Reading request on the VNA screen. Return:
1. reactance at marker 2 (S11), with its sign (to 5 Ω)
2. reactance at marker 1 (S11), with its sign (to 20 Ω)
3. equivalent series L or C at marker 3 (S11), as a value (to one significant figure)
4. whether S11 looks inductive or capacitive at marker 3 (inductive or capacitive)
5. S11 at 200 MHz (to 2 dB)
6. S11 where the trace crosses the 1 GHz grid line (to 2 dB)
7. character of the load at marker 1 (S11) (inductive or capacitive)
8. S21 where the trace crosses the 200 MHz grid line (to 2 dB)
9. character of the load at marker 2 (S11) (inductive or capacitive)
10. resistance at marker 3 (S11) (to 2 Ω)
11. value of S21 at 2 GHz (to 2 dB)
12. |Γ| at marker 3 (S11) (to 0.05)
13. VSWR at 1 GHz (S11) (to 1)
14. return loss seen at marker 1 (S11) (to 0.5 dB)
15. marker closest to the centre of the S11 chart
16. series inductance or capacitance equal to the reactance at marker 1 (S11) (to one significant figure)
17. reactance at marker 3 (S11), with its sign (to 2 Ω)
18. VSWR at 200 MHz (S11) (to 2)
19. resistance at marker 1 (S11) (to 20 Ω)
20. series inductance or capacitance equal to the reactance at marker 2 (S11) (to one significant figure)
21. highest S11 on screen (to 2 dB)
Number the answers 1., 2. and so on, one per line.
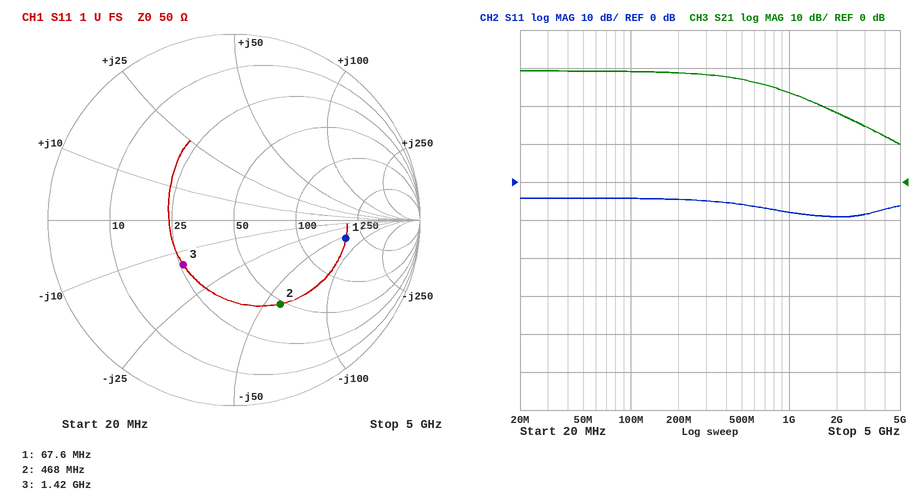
1. -60 Ω
2. -60 Ω
3. 8 pF
4. capacitive
5. -4 dB
6. -8 dB
7. capacitive
8. 28 dB
9. capacitive
10. 26 Ω
11. 18 dB
12. 0.35
13. 2
14. 4.5 dB
15. marker 3
16. 40 pF
17. -14 Ω
18. 4
19. 180 Ω
20. 6 pF
21. -4 dB
